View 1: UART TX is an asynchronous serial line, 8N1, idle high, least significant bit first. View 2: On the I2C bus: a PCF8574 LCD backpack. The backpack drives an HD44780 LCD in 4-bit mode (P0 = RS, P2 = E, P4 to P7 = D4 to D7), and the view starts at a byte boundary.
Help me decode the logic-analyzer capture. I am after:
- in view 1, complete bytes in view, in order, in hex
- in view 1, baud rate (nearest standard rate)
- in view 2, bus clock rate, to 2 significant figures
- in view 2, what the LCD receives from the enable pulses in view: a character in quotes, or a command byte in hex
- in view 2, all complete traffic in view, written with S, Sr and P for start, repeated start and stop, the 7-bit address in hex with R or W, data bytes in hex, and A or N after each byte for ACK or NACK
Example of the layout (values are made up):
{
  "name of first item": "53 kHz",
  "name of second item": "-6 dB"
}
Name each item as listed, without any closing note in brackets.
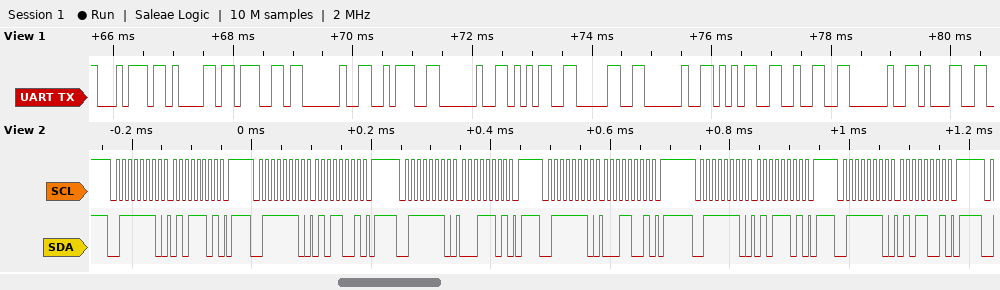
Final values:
{
  "in view 1, complete bytes in view, in order, in hex": "74 61 67 20 3A 20 35 30 20 35 32 20 31",
  "in view 1, baud rate": "9600 baud",
  "in view 2, bus clock rate, to 2 significant figures": "100 kHz",
  "in view 2, what the LCD receives from the enable pulses in view: a character in quotes, or a command byte in hex": "'Q'",
  "in view 2, all complete traffic in view, written with S, Sr and P for start, repeated start and stop, the 7-bit address in hex with R or W, data bytes in hex, and A or N after each byte for ACK or NACK": "S 3FW A 5D A P S 3FW A 59 A P S 3FW A 1D A P S 3FW A 19 A P S 3FW A 5D A P S 3FW A 59 A P"
}
